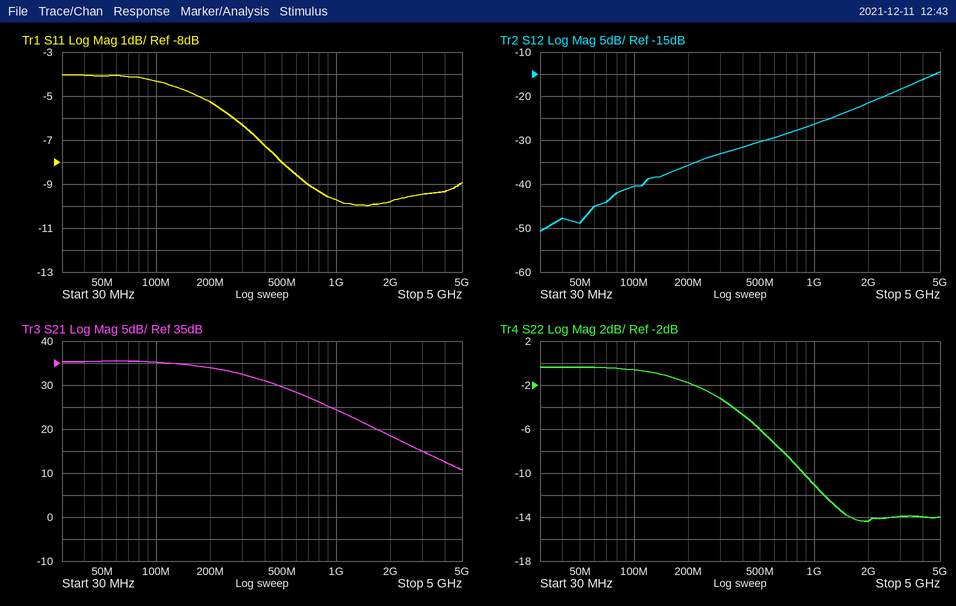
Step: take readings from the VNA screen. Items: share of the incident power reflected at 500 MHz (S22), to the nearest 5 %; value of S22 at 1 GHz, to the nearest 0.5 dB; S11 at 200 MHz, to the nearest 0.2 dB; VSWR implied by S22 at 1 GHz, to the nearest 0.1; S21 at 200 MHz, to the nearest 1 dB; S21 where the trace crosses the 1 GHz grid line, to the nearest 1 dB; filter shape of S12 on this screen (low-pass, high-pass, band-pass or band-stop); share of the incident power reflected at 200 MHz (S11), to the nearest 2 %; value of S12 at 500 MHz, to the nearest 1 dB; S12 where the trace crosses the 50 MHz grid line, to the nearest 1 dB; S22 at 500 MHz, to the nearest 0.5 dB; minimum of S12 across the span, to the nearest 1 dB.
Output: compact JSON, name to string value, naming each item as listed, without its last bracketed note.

{"share of the incident power reflected at 500 MHz (S22), to the nearest 5 %": "25 %", "value of S22 at 1 GHz, to the nearest 0.5 dB": "-11.0 dB", "S11 at 200 MHz, to the nearest 0.2 dB": "-5.2 dB", "VSWR implied by S22 at 1 GHz, to the nearest 0.1": "1.8", "S21 at 200 MHz, to the nearest 1 dB": "34 dB", "S21 where the trace crosses the 1 GHz grid line, to the nearest 1 dB": "24 dB", "filter shape of S12 on this screen": "high-pass", "share of the incident power reflected at 200 MHz (S11), to the nearest 2 %": "30 %", "value of S12 at 500 MHz, to the nearest 1 dB": "-30 dB", "S12 where the trace crosses the 50 MHz grid line, to the nearest 1 dB": "-49 dB", "S22 at 500 MHz, to the nearest 0.5 dB": "-6.0 dB", "minimum of S12 across the span, to the nearest 1 dB": "-51 dB"}
